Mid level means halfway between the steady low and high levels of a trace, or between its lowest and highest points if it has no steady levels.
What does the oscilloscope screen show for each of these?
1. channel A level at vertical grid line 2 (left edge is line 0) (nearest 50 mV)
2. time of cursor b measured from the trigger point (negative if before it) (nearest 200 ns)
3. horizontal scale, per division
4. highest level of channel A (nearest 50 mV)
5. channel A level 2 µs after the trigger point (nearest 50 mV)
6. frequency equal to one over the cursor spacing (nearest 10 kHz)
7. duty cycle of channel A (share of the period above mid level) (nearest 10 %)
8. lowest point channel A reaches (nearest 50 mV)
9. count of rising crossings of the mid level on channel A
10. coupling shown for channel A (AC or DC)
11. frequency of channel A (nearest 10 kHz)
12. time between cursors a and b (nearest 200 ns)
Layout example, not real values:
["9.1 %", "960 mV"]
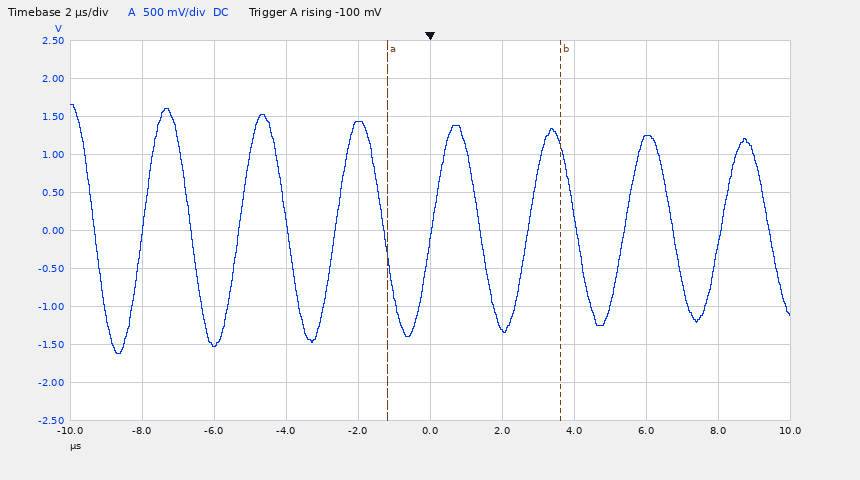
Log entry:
["-1.50 V", "+3.6 µs", "2 µs", "1.65 V", "-1.30 V", "210 kHz", "50 %", "-1.60 V", "7", "DC", "370 kHz", "4.8 µs"]
